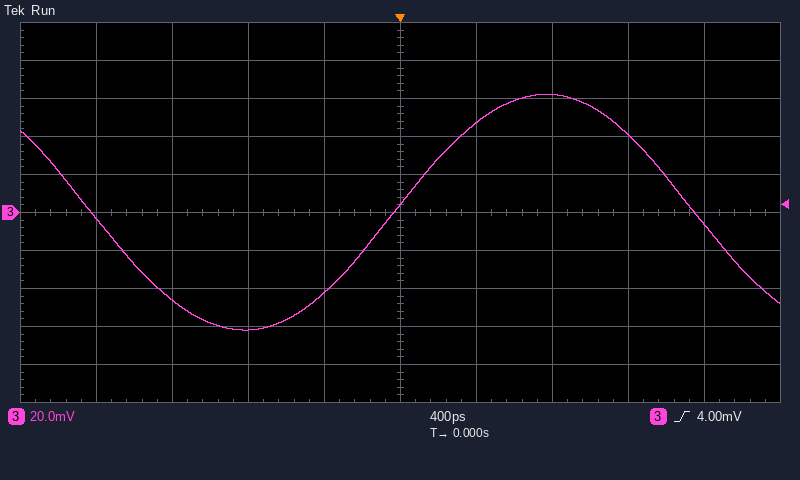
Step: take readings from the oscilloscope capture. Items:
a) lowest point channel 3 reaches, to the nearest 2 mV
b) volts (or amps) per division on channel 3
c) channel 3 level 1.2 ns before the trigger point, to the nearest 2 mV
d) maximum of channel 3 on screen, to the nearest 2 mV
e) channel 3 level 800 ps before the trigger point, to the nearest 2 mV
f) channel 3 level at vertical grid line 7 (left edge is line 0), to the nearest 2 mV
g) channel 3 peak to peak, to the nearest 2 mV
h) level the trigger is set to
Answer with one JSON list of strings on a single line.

["-62 mV", "20 mV", "-46 mV", "62 mV", "-62 mV", "62 mV", "124 mV", "4.00 mV"]
